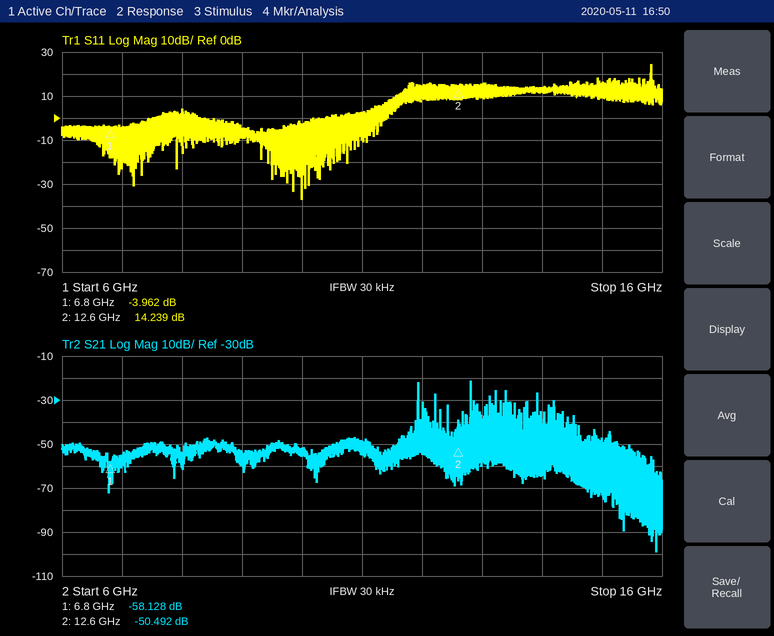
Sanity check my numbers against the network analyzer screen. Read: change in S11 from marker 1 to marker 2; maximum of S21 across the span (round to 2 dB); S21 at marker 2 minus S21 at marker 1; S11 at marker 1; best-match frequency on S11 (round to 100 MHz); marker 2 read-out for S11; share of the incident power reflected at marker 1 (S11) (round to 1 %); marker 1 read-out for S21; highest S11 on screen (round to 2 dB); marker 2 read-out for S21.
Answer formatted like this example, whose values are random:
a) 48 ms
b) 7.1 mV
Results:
a) 18.201 dB
b) -22 dB
c) 7.636 dB
d) -3.962 dB
e) 10.0 GHz
f) 14.239 dB
g) 40 %
h) -58.128 dB
i) 24 dB
j) -50.492 dB
